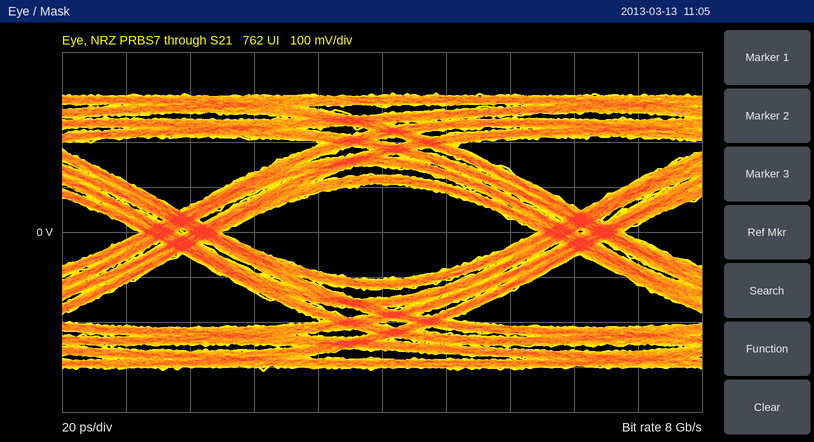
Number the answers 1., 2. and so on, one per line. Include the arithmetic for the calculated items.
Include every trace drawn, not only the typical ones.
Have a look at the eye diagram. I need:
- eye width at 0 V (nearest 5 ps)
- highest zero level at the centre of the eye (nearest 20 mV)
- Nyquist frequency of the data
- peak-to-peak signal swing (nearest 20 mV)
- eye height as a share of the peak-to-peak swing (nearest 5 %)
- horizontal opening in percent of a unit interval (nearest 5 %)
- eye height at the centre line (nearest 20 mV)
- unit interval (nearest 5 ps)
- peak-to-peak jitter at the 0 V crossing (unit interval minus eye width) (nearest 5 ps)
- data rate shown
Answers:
1. 100 ps
2. -100 mV
3. 4 GHz
4. 620 mV
5. 220 mV / 620 mV ≈ 35 %
6. 100 ps / 125 ps ≈ 80 %
7. 220 mV
8. 125 ps
9. 25 ps
10. 8 Gb/s
